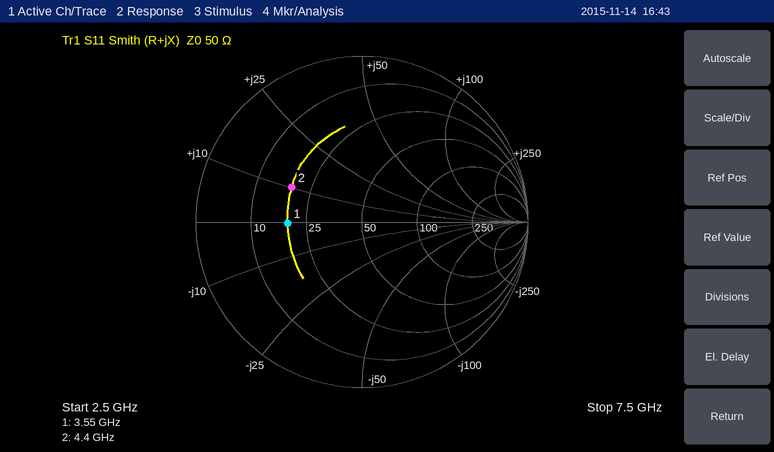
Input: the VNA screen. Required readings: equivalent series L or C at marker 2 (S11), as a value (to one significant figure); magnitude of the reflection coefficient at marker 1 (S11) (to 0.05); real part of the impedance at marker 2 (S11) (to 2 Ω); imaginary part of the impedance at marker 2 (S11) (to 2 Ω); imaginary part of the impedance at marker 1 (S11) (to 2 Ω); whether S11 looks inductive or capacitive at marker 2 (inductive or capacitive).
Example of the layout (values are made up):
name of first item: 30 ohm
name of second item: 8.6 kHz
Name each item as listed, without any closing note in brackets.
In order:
equivalent series L or C at marker 2 (S11), as a value: 400 pH
magnitude of the reflection coefficient at marker 1 (S11): 0.45
real part of the impedance at marker 2 (S11): 18 Ω
imaginary part of the impedance at marker 2 (S11): +10 Ω
imaginary part of the impedance at marker 1 (S11): 0 Ω
whether S11 looks inductive or capacitive at marker 2: inductive
